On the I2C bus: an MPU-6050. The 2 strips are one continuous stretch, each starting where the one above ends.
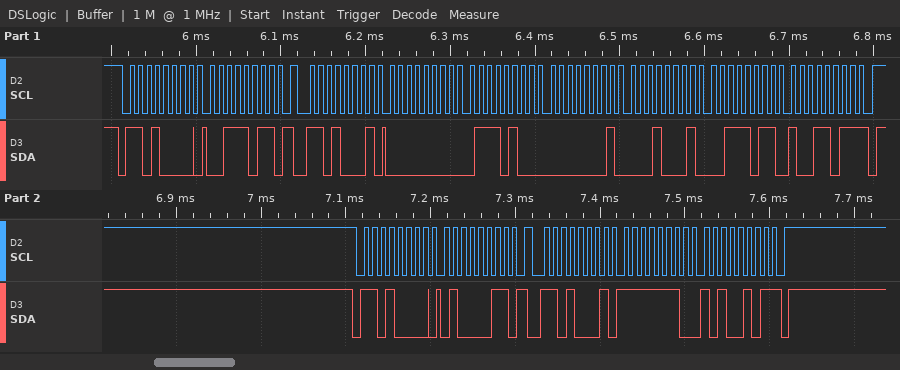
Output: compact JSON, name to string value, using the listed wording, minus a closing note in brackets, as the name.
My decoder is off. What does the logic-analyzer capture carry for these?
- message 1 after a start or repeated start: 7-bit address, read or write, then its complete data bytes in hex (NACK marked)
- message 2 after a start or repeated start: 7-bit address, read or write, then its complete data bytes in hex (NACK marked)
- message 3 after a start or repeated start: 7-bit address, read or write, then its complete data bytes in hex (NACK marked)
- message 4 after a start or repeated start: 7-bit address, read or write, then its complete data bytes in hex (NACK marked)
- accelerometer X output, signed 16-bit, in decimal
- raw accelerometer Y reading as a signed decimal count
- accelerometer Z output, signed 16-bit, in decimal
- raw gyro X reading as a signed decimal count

{"message 1 after a start or repeated start: 7-bit address, read or write, then its complete data bytes in hex": "0x68 write: 3B", "message 2 after a start or repeated start: 7-bit address, read or write, then its complete data bytes in hex": "0x68 read: 00 74 01 11 3B 9B NACK", "message 3 after a start or repeated start: 7-bit address, read or write, then its complete data bytes in hex": "0x68 write: 43", "message 4 after a start or repeated start: 7-bit address, read or write, then its complete data bytes in hex": "0x68 read: FE A5 NACK", "accelerometer X output, signed 16-bit, in decimal": "116", "raw accelerometer Y reading as a signed decimal count": "273", "accelerometer Z output, signed 16-bit, in decimal": "15259", "raw gyro X reading as a signed decimal count": "-347"}
